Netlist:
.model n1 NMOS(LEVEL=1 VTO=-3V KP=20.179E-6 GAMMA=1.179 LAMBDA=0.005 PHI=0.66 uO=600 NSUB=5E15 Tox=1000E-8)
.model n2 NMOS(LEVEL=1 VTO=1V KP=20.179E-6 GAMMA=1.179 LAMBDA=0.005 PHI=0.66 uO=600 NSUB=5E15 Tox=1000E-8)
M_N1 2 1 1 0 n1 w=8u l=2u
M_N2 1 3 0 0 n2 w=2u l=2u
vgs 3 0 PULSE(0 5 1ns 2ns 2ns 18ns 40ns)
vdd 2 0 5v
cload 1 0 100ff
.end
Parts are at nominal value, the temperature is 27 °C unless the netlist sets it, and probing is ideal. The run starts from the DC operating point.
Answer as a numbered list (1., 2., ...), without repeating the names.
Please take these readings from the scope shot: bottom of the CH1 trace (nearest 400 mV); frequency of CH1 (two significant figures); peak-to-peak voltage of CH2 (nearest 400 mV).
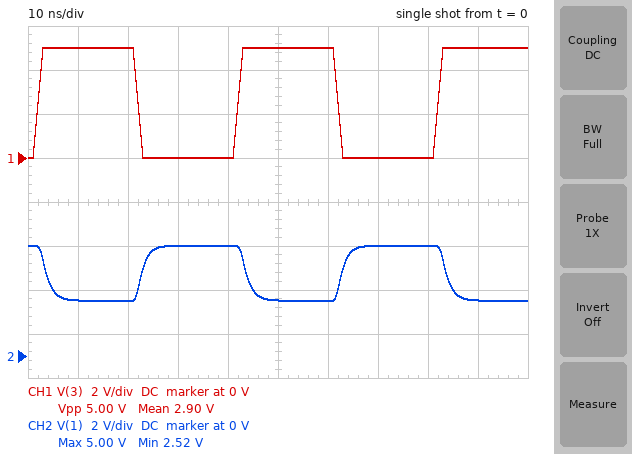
1. 0 V
2. 25 MHz
3. 2.4 V
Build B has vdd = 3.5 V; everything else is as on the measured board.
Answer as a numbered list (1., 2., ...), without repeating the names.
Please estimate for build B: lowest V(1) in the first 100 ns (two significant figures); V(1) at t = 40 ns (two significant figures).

1. 2.3 V
2. 3.5 V
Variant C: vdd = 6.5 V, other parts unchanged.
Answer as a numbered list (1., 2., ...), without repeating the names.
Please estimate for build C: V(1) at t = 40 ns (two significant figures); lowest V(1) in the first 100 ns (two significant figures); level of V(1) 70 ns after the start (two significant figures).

1. 6.5 V
2. 2.5 V
3. 6.4 V
